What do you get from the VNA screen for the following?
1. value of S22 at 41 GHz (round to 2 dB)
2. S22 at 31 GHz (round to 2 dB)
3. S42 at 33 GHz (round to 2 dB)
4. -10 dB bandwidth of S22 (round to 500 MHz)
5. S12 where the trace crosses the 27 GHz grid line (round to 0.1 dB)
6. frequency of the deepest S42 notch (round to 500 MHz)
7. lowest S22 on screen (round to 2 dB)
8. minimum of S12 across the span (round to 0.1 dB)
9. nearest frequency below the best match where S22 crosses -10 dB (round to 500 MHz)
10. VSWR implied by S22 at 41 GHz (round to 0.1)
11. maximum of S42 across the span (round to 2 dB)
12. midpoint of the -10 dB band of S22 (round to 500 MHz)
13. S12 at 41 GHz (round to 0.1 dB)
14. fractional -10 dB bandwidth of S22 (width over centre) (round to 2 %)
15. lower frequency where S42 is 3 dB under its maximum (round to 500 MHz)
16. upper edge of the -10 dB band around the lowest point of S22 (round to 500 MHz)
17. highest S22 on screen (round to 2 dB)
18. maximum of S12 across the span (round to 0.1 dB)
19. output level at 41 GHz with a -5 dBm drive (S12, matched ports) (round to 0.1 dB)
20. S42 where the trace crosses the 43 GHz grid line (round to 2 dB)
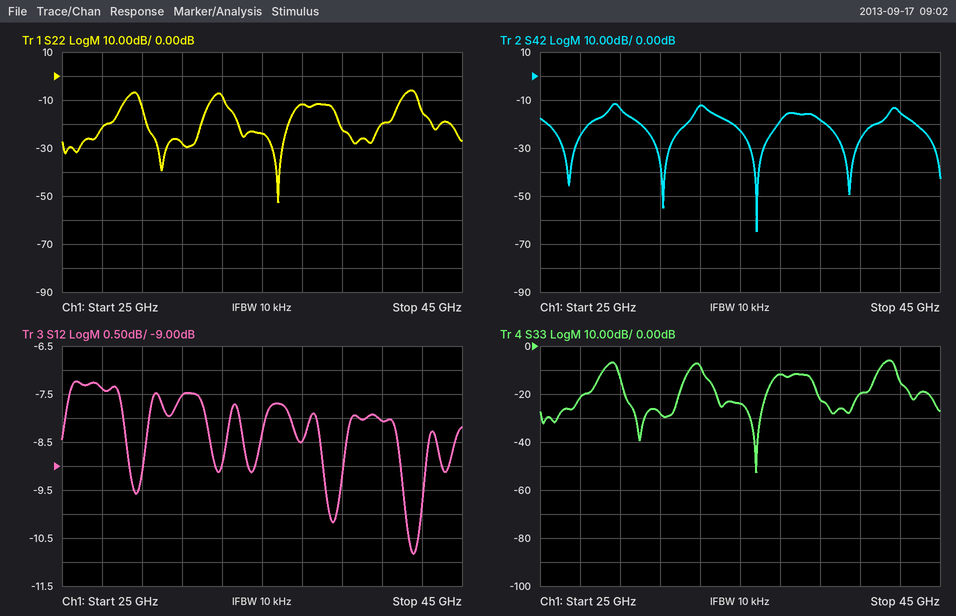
-20 dB
-28 dB
-12 dB
9.0 GHz
-7.4 dB
36.0 GHz
-52 dB
-10.8 dB
33.0 GHz
1.2
-12 dB
37.5 GHz
-8.1 dB
24 %
28.5 GHz
42.0 GHz
-6 dB
-7.2 dB
-13.1 dBm
-16 dB
